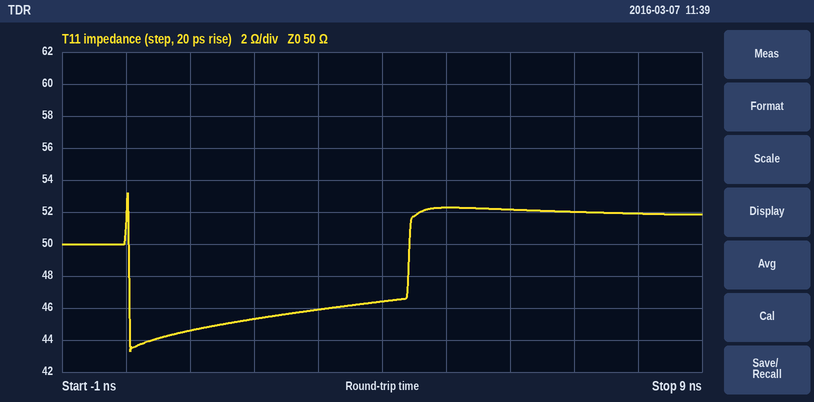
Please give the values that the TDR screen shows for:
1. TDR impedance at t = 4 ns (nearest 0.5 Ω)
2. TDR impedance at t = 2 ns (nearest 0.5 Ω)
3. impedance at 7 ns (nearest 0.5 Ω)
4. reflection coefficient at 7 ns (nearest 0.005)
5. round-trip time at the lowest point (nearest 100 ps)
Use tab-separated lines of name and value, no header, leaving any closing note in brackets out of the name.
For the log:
TDR impedance at t = 4 ns	46.5 Ω
TDR impedance at t = 2 ns	45.5 Ω
impedance at 7 ns	52.0 Ω
reflection coefficient at 7 ns	+0.020
round-trip time at the lowest point	100 ps
